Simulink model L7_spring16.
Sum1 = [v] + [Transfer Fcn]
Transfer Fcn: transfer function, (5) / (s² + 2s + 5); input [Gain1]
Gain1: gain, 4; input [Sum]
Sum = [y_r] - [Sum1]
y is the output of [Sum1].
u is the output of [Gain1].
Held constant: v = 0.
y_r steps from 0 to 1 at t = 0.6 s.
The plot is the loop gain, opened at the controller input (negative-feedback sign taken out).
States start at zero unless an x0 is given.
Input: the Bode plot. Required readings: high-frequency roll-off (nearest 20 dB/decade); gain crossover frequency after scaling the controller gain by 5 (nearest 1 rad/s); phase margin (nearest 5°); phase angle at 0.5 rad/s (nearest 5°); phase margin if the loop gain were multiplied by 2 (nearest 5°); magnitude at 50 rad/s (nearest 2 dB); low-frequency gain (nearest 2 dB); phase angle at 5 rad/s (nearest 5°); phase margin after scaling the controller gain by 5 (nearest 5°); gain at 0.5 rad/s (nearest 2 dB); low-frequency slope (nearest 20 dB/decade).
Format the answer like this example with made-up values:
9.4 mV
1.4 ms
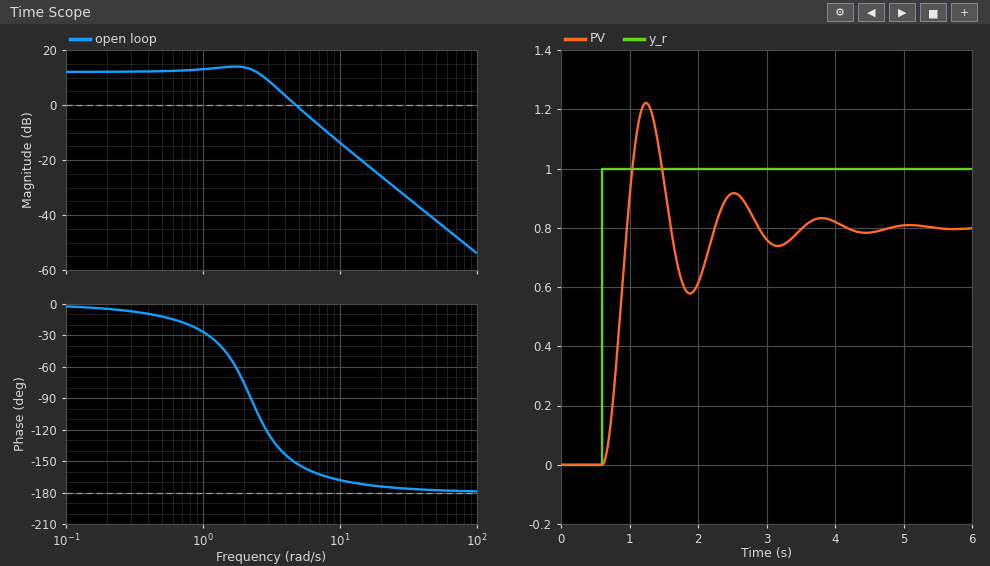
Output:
-40 dB/decade
10 rad/s
30°
-10°
20°
-42 dB
12 dB
-155°
10°
12 dB
0 dB/decade
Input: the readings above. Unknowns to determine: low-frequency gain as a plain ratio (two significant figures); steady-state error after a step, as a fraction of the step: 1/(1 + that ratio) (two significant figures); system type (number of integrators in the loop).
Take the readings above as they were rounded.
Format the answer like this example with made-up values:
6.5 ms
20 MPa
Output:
4.0
0.20
0
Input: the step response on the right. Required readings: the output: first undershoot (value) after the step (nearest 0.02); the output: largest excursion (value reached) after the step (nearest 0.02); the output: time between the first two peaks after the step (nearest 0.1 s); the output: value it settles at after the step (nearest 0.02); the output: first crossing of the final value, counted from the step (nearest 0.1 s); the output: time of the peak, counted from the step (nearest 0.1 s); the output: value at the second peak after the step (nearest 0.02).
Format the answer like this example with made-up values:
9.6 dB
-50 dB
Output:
0.58
1.22
1.3 s
0.80
0.4 s
0.6 s
0.92
